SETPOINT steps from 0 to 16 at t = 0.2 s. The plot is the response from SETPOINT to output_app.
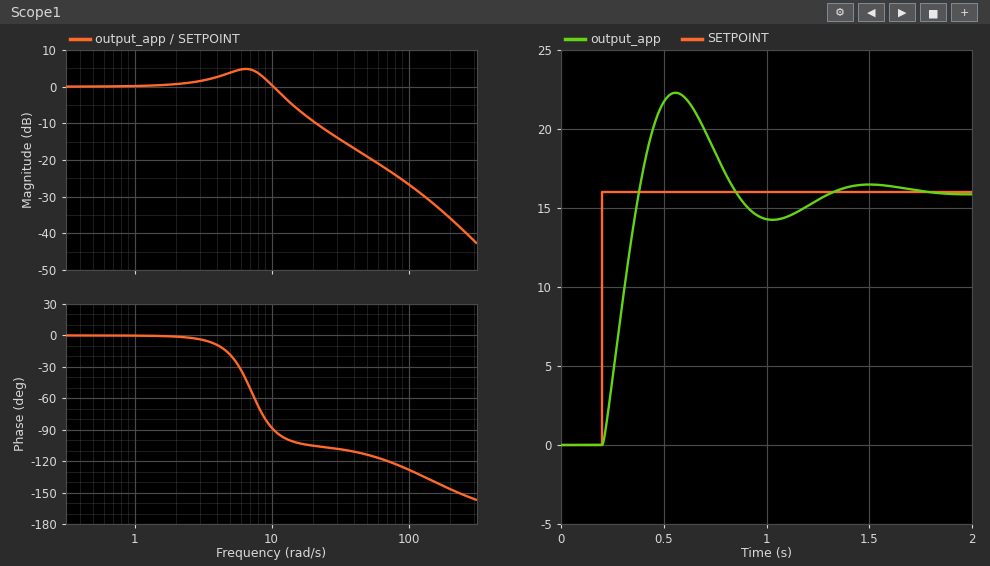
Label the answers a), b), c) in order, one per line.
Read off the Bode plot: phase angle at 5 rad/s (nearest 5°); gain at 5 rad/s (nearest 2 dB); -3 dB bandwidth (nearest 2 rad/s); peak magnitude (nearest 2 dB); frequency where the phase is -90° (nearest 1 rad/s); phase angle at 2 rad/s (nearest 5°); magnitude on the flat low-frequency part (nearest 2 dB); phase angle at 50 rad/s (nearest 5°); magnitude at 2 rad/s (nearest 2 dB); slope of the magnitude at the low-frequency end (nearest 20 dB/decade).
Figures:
a) -20°
b) 4 dB
c) 12 rad/s
d) 4 dB
e) 10 rad/s
f) 0°
g) 0 dB
h) -115°
i) 0 dB
j) 0 dB/decade
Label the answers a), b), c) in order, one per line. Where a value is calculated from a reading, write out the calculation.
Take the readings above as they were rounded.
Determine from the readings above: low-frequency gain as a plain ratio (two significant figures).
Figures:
a) 10^(0 / 20) = 1.0
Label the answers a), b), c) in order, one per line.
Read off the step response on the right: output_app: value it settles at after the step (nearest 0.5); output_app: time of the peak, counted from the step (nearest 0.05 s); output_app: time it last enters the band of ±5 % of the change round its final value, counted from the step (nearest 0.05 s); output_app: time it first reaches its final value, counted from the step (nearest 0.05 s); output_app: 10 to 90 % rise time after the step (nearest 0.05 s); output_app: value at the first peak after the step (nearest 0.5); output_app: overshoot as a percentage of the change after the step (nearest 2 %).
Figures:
a) 16.0
b) 0.35 s
c) 1.00 s
d) 0.20 s
e) 0.15 s
f) 22.5
g) 40 %
